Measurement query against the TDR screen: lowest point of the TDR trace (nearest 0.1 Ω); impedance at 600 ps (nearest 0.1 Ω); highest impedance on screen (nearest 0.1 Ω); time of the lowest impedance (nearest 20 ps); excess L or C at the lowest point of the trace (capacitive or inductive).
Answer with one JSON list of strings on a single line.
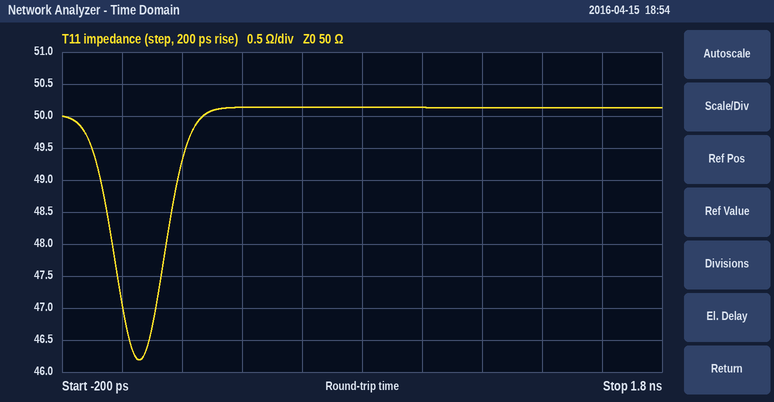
["46.2 Ω", "50.1 Ω", "50.1 Ω", "60 ps", "capacitive"]
